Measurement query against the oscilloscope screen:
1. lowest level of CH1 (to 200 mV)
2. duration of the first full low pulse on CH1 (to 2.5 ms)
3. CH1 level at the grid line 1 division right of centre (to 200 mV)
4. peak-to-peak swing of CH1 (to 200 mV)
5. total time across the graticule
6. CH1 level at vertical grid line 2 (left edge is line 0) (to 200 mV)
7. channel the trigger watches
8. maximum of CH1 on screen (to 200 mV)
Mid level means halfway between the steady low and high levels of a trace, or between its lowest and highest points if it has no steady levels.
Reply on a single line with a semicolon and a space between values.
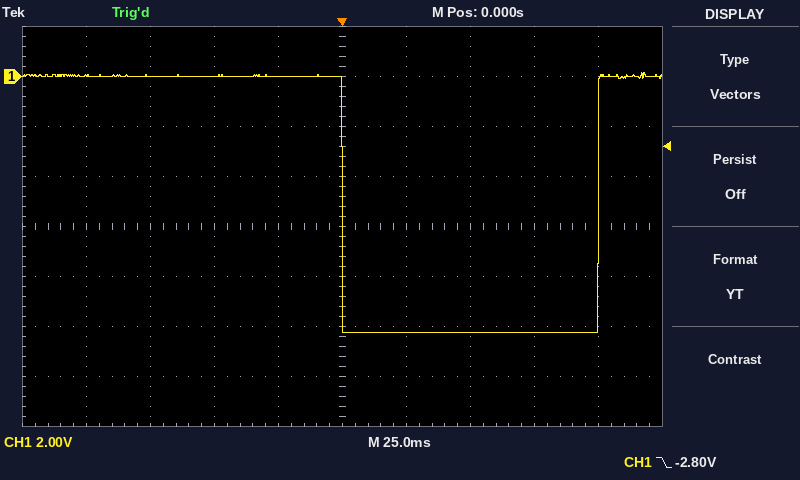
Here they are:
-10.2 V; 100.0 ms; -10.2 V; 10.4 V; 250 ms; 0.0 V; CH1; 200 mV
